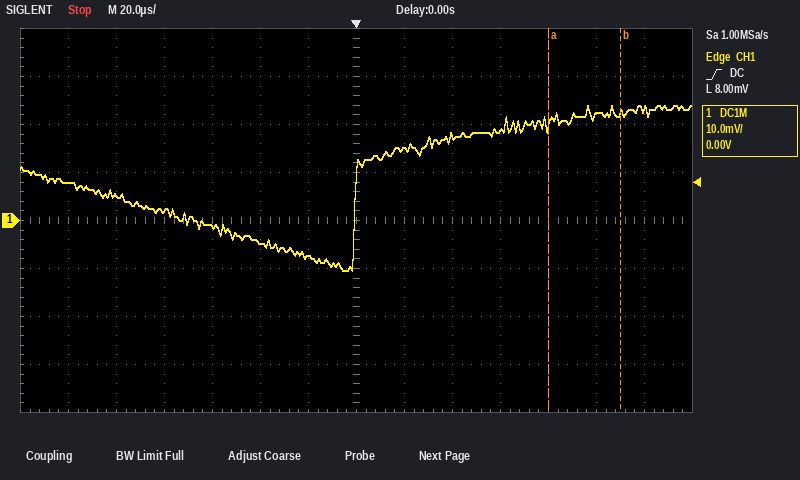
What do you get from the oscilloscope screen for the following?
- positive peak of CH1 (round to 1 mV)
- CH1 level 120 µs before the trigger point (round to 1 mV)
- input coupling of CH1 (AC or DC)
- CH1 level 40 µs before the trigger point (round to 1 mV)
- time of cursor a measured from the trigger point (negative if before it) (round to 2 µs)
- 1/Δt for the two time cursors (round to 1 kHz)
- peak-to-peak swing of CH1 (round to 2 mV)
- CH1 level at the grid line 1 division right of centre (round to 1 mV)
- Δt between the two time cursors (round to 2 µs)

24 mV
8 mV
DC
-5 mV
+80 µs
33 kHz
34 mV
15 mV
30 µs
